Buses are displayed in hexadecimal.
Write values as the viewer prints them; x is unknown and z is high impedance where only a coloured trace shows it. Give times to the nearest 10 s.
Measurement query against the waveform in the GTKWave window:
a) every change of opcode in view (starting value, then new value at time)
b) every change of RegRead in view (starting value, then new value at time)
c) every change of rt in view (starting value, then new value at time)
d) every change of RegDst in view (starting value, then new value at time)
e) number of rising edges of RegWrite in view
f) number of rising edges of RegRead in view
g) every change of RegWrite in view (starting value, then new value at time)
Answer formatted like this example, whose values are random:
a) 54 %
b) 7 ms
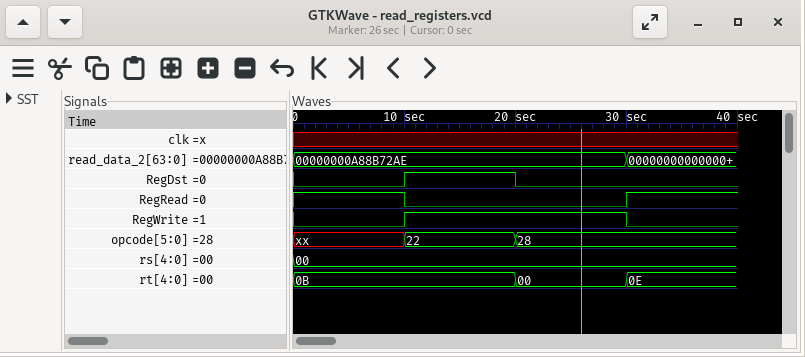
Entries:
a) xx, 22 at 10 s, 28 at 20 s
b) 1, 0 at 10 s, 1 at 30 s
c) 0B, 00 at 20 s, 0E at 30 s
d) 0, 1 at 10 s, 0 at 20 s
e) 1
f) 1
g) 0, 1 at 10 s, 0 at 30 s
